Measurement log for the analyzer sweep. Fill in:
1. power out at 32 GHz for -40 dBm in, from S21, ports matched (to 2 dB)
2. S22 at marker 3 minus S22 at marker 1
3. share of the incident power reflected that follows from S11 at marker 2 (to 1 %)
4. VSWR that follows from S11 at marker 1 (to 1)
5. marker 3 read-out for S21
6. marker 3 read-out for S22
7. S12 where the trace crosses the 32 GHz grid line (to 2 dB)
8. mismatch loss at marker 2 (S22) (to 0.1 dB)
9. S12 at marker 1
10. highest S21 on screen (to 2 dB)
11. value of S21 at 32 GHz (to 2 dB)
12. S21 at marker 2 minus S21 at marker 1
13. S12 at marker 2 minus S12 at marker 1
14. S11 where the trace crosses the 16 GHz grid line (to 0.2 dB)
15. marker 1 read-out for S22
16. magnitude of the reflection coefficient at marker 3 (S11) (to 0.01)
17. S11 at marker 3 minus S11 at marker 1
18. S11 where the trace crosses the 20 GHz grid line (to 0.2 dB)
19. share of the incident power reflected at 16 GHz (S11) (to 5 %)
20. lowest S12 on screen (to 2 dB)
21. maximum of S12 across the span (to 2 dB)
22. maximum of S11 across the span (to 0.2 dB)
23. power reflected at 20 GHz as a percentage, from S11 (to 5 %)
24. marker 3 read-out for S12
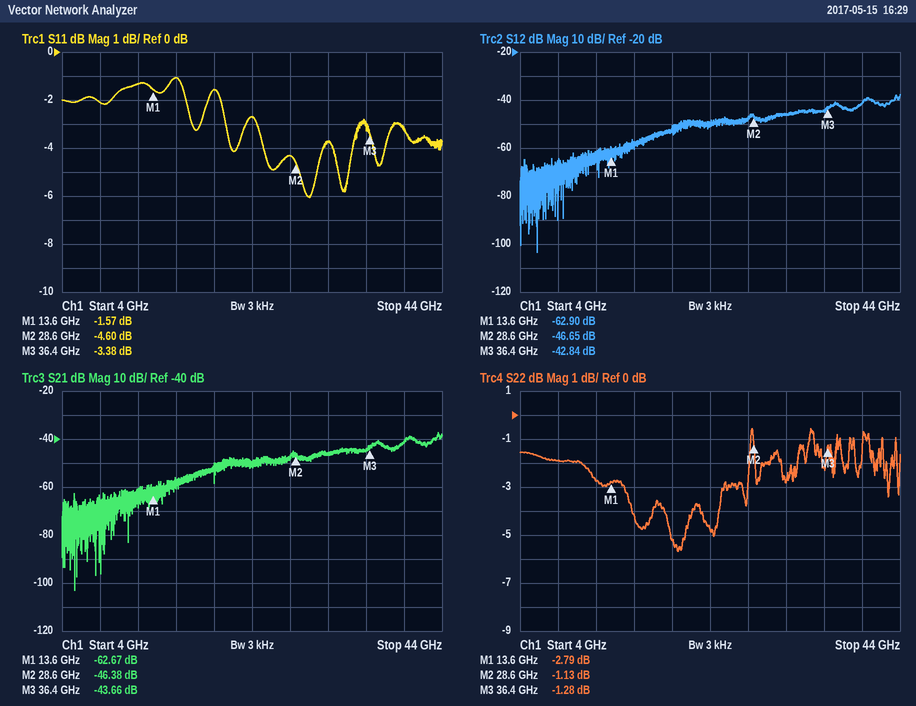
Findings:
-86 dBm
1.51 dB
35 %
11
-43.66 dB
-1.28 dB
-46 dB
6.4 dB
-62.90 dB
-38 dB
-46 dB
16.29 dB
16.25 dB
-1.0 dB
-2.79 dB
0.68
-1.81 dB
-1.6 dB
80 %
-104 dB
-38 dB
-1.0 dB
70 %
-42.84 dB
